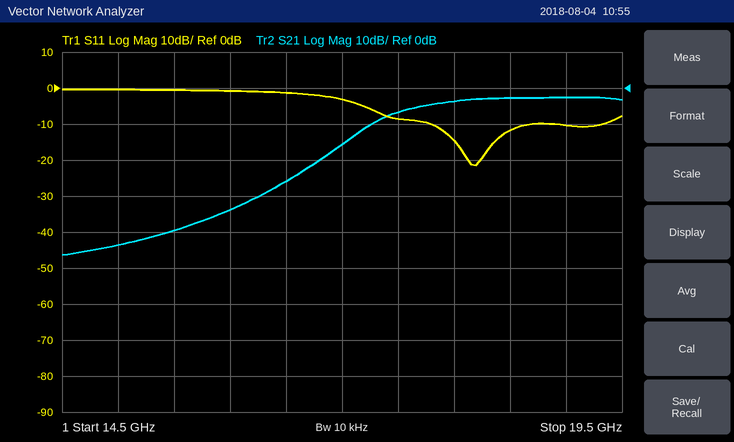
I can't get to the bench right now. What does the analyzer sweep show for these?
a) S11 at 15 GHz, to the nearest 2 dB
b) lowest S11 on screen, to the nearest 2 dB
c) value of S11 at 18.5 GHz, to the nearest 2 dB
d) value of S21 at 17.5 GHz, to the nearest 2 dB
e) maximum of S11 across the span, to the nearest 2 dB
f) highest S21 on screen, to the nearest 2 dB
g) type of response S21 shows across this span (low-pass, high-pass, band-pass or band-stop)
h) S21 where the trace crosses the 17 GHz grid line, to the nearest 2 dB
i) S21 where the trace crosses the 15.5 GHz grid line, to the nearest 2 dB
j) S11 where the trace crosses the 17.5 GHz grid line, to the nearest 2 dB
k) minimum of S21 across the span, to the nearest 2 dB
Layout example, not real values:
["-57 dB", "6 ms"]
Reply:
["0 dB", "-22 dB", "-12 dB", "-6 dB", "0 dB", "-2 dB", "high-pass", "-16 dB", "-40 dB", "-8 dB", "-46 dB"]
